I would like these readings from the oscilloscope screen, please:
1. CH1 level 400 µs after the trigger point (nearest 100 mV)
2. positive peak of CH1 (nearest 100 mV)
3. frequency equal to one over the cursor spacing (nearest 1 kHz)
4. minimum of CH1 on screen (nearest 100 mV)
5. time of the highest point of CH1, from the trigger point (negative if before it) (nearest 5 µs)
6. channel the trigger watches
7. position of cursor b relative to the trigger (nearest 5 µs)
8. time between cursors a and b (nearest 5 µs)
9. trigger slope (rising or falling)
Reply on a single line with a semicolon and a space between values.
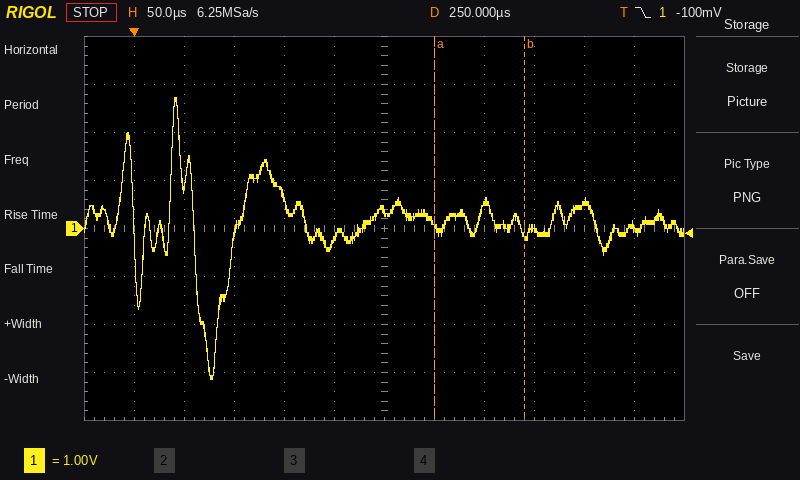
0.0 V; 2.7 V; 11 kHz; -3.1 V; +40 µs; CH1; +390 µs; 90 µs; falling
